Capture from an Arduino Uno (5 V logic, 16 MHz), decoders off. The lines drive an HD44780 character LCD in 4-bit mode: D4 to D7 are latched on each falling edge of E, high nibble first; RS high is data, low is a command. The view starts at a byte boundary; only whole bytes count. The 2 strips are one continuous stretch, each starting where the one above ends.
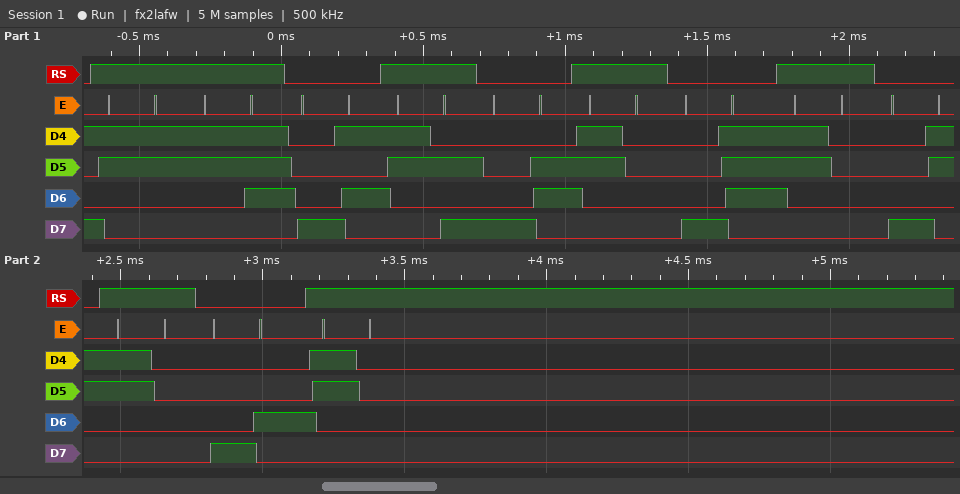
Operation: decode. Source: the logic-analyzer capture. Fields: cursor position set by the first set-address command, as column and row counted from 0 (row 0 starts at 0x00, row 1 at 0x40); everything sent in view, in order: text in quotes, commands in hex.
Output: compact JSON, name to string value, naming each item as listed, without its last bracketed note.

{"cursor position set by the first set-address command, as column and row counted from 0": "column 5, row 0", "everything sent in view, in order: text in quotes, commands in hex": "\"37\" 0x85 \":\" 0x86 \"0\" 0x87 \"0\" 0x83 \"0\" 0x84 \"0\""}
